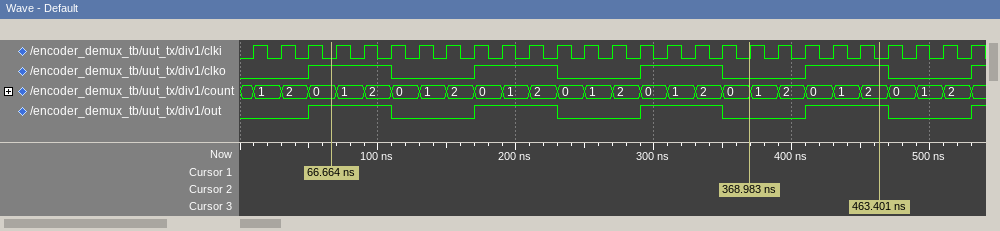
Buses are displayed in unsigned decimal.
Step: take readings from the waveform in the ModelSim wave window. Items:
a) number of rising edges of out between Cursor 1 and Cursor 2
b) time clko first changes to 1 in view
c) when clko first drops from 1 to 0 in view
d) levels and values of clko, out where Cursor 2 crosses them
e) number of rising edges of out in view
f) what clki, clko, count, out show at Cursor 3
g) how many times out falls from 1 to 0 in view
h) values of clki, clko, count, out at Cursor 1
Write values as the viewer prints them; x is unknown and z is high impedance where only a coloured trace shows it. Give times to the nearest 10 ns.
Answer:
2
50 ns
110 ns
clko=0, out=0
5
clki=0, clko=1, count=2, out=1
4
clki=0, clko=1, count=0, out=1
